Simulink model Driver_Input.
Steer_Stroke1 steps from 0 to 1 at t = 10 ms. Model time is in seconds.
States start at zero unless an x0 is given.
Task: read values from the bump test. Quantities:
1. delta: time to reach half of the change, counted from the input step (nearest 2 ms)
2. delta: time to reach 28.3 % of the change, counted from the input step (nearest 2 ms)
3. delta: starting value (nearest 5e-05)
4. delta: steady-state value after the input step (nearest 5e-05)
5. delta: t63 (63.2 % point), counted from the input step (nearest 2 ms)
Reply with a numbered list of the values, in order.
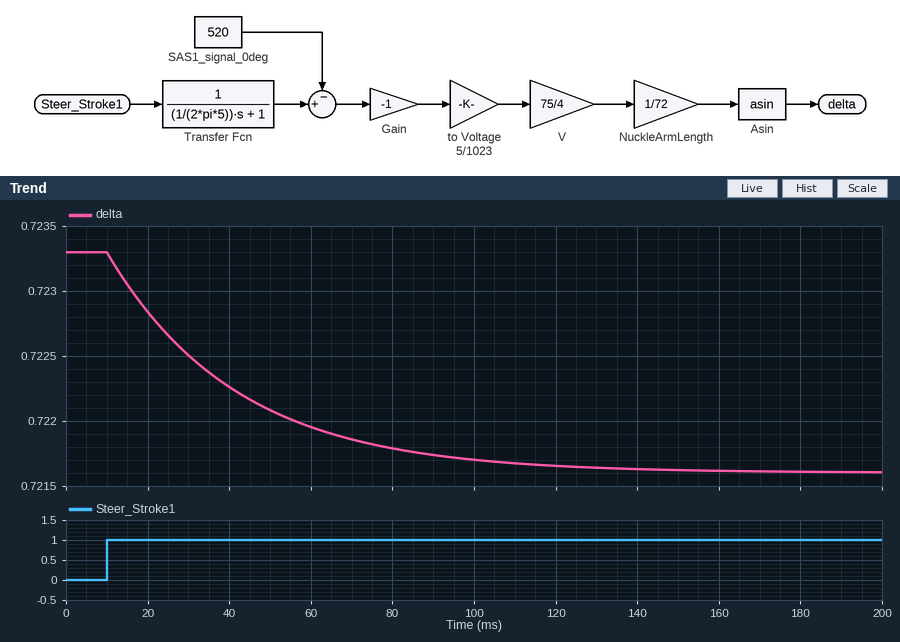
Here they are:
1. 22 ms
2. 10 ms
3. 0.72330
4. 0.72160
5. 32 ms
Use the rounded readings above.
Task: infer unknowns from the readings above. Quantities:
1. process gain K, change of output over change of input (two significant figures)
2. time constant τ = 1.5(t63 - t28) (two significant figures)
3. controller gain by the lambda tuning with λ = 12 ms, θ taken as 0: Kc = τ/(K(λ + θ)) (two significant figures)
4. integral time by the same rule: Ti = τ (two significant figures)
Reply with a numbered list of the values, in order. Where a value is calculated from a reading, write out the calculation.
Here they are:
1. (0.7216 - 0.7233) / 1 = -0.0017
2. 1.5 × (32 - 10) = 33 ms
3. 33 / (-0.0017 × (12 + 0)) = -1600
4. 33 ms
